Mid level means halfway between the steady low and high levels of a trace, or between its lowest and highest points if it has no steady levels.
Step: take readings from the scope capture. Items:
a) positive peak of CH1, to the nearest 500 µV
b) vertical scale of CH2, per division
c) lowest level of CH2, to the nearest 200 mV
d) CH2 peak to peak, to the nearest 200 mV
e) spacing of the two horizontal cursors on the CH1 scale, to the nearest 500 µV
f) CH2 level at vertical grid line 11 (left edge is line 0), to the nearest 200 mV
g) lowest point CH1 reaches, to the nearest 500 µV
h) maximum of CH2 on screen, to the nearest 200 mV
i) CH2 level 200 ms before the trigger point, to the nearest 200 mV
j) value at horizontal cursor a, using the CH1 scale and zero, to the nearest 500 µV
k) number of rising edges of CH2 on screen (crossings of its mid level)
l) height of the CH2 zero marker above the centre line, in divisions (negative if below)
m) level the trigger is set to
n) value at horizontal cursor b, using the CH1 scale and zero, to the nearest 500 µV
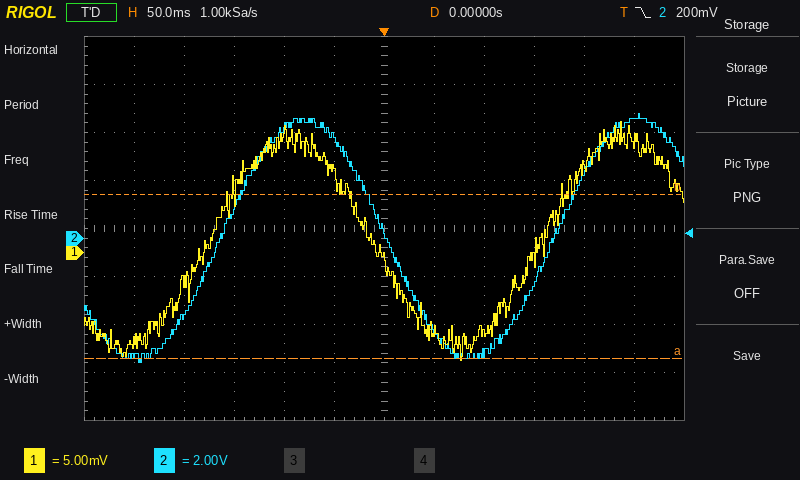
13.5 mV
2 V
-5.2 V
10.4 V
17.0 mV
5.0 V
-11.0 mV
5.2 V
-3.2 V
-11.0 mV
2
-0.2 div
200 mV
6.0 mV
